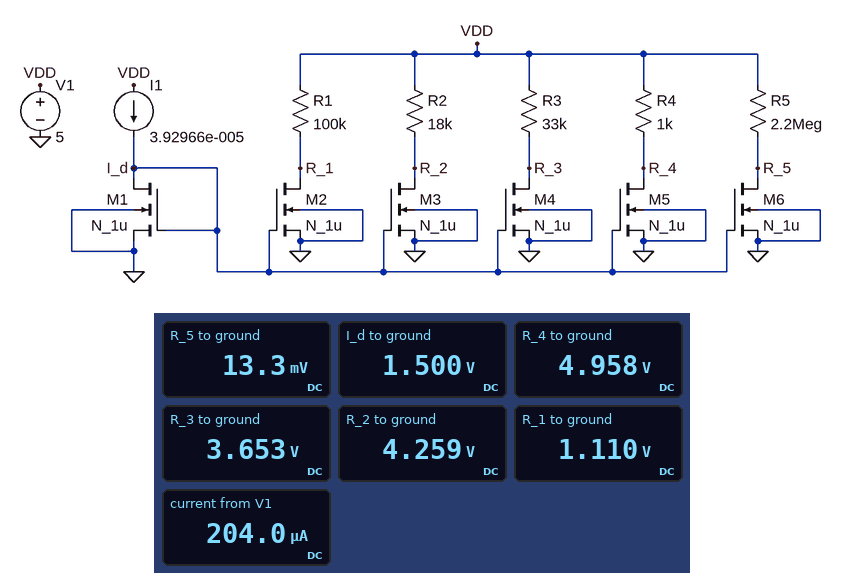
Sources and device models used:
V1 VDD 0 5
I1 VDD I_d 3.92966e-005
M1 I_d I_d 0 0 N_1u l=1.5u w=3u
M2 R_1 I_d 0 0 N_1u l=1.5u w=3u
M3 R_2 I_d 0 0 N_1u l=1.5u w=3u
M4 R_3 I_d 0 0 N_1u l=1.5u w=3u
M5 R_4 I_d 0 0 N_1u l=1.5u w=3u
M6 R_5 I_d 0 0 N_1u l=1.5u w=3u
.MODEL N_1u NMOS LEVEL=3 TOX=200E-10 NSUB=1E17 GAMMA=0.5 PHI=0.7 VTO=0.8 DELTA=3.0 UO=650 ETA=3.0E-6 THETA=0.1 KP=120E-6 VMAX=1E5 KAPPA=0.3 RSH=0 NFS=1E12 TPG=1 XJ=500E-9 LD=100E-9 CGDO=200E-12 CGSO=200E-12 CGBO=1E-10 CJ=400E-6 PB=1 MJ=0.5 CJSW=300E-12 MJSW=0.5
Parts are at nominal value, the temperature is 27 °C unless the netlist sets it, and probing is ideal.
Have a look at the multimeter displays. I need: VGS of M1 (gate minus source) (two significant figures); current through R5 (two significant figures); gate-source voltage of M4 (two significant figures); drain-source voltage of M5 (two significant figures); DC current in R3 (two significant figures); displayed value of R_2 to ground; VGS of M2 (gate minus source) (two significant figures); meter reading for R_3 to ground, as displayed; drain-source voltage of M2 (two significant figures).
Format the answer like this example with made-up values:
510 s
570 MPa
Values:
1.5 V
2.3 µA
1.5 V
5.0 V
41 µA
4.259 V
1.5 V
3.653 V
1.1 V
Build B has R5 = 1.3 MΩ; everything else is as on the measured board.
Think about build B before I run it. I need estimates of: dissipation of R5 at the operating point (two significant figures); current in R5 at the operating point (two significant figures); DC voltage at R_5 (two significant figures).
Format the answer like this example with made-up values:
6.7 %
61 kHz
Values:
19 µW
3.8 µA
23 mV
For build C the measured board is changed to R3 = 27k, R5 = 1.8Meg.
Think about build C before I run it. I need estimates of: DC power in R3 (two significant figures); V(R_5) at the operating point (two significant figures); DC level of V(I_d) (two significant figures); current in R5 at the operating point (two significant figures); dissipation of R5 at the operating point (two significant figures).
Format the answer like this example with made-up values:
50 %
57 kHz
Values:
45 µW
16 mV
1.5 V
2.8 µA
14 µW
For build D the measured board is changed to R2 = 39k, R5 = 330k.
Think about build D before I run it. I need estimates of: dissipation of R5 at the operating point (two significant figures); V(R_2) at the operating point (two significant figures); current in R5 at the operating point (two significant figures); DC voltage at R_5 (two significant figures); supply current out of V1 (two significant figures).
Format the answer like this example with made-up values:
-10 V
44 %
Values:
73 µW
3.4 V
15 µA
99 mV
220 µA
